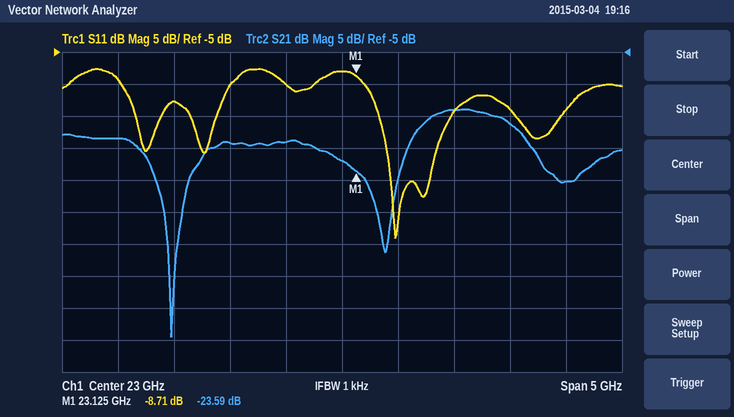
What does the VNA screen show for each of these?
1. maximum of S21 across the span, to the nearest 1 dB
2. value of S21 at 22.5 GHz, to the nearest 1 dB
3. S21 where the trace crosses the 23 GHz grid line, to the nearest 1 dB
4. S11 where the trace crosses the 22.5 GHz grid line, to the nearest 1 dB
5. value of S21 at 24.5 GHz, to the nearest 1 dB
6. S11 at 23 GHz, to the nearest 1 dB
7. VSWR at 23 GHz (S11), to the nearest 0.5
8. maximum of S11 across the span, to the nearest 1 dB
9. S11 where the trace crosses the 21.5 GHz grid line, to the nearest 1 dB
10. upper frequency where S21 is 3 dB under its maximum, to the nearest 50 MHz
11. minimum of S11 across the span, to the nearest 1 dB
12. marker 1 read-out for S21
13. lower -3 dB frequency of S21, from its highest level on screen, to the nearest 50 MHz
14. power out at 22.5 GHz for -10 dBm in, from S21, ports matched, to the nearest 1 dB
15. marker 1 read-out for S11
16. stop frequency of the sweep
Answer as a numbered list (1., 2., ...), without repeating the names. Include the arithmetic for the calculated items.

1. -14 dB
2. -19 dB
3. -22 dB
4. -10 dB
5. -16 dB
6. -8 dB
7. |Γ| = 10^(-8/20) = 0.3981; VSWR = (1 + 0.3981)/(1 − 0.3981) ≈ 2.32, so 2.5 to the nearest 0.5
8. -8 dB
9. -13 dB
10. 24.55 GHz
11. -34 dB
12. -23.59 dB
13. 23.70 GHz
14. -10 dBm + (-19 dB) = -29 dBm
15. -8.71 dB
16. 25.5 GHz
